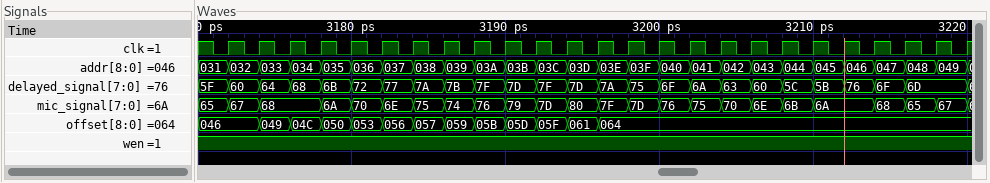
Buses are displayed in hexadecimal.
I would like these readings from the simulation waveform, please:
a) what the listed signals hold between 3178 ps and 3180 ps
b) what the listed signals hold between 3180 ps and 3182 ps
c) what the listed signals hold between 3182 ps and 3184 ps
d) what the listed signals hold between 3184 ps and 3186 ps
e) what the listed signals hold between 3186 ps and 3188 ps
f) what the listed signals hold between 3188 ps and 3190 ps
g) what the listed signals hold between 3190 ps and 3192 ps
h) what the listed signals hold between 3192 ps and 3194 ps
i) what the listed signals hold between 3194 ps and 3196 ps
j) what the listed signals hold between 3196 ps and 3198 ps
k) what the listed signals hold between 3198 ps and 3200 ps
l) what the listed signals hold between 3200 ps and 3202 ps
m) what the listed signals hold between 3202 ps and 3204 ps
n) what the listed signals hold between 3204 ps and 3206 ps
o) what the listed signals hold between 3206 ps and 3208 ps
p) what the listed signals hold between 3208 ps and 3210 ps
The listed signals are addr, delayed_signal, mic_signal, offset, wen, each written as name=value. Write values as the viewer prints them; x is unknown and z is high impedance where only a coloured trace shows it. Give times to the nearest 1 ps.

addr=035, delayed_signal=6B, mic_signal=6A, offset=050, wen=1
addr=036, delayed_signal=72, mic_signal=70, offset=053, wen=1
addr=037, delayed_signal=77, mic_signal=6E, offset=056, wen=1
addr=038, delayed_signal=7A, mic_signal=75, offset=057, wen=1
addr=039, delayed_signal=7B, mic_signal=74, offset=059, wen=1
addr=03A, delayed_signal=7F, mic_signal=76, offset=05B, wen=1
addr=03B, delayed_signal=7D, mic_signal=79, offset=05D, wen=1
addr=03C, delayed_signal=7F, mic_signal=7D, offset=05F, wen=1
addr=03D, delayed_signal=7D, mic_signal=80, offset=061, wen=1
addr=03E, delayed_signal=7A, mic_signal=7F, offset=064, wen=1
addr=03F, delayed_signal=75, mic_signal=7D, offset=064, wen=1
addr=040, delayed_signal=6F, mic_signal=76, offset=064, wen=1
addr=041, delayed_signal=6A, mic_signal=75, offset=064, wen=1
addr=042, delayed_signal=63, mic_signal=70, offset=064, wen=1
addr=043, delayed_signal=60, mic_signal=6E, offset=064, wen=1
addr=044, delayed_signal=5C, mic_signal=6B, offset=064, wen=1
